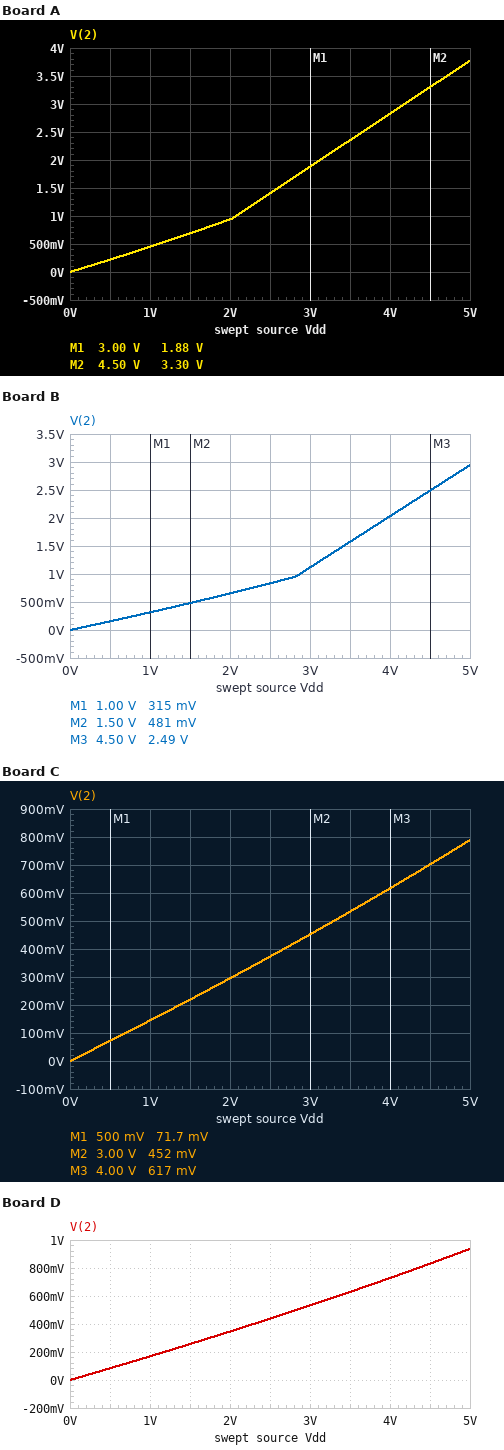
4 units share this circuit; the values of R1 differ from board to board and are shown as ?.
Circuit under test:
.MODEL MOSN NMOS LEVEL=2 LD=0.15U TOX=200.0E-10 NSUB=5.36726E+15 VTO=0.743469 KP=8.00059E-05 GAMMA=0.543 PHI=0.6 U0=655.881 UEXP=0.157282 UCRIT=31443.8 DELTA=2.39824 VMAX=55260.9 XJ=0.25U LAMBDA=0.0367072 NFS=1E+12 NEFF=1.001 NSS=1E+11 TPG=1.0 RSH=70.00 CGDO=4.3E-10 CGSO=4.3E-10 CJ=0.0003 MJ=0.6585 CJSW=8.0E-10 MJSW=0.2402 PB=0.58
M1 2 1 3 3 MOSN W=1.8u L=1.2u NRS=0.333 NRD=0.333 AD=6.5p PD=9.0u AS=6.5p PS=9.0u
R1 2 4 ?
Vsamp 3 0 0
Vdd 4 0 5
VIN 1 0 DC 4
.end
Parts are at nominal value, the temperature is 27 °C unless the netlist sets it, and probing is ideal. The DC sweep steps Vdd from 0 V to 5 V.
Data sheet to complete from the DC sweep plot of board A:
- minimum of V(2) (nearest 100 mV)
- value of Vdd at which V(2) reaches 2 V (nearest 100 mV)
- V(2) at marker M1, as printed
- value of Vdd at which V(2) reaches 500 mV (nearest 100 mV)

0 V
3.1 V
1.88 V
1.1 V
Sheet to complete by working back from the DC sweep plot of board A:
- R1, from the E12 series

3.9 kΩ
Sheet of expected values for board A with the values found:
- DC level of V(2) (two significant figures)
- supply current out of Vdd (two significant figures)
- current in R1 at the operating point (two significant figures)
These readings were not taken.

3.8 V
310 µA
310 µA
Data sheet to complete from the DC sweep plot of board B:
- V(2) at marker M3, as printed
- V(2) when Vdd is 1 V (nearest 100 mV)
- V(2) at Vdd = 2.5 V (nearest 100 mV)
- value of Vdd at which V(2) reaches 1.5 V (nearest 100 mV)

2.49 V
300 mV
800 mV
3.4 V
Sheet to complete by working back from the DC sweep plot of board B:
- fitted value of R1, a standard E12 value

6.8 kΩ
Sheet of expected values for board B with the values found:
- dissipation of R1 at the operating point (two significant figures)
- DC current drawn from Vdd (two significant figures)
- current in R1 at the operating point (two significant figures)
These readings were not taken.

620 µW
300 µA
300 µA
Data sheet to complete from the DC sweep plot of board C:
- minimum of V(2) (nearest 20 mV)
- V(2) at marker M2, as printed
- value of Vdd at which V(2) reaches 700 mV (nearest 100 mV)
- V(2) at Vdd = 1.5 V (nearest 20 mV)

0 V
452 mV
4.5 V
220 mV
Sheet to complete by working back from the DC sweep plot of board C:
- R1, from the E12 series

18 kΩ
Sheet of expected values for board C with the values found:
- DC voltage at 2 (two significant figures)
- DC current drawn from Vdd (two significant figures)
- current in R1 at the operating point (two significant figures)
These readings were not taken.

790 mV
230 µA
230 µA
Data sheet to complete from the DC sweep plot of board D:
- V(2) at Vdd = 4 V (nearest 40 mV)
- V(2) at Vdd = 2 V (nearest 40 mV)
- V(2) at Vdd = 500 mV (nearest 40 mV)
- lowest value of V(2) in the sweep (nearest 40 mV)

720 mV
360 mV
80 mV
0 V
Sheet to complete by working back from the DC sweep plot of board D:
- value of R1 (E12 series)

15 kΩ
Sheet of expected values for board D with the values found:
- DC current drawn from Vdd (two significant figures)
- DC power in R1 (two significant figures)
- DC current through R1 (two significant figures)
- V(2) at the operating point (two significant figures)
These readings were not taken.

270 µA
1.1 mW
270 µA
940 mV
